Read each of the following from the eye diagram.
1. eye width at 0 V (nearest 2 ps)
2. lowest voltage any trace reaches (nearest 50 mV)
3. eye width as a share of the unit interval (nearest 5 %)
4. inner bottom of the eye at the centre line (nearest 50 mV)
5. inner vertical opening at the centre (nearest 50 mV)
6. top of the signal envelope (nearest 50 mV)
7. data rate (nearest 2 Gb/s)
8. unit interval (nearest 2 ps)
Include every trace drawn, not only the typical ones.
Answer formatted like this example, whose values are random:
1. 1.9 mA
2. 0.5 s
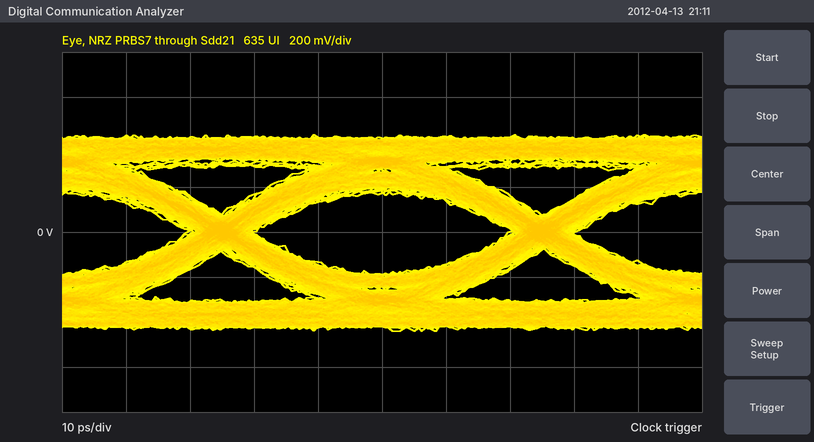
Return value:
1. 40 ps
2. -450 mV
3. 80 %
4. -200 mV
5. 350 mV
6. 450 mV
7. 20 Gb/s
8. 50 ps
